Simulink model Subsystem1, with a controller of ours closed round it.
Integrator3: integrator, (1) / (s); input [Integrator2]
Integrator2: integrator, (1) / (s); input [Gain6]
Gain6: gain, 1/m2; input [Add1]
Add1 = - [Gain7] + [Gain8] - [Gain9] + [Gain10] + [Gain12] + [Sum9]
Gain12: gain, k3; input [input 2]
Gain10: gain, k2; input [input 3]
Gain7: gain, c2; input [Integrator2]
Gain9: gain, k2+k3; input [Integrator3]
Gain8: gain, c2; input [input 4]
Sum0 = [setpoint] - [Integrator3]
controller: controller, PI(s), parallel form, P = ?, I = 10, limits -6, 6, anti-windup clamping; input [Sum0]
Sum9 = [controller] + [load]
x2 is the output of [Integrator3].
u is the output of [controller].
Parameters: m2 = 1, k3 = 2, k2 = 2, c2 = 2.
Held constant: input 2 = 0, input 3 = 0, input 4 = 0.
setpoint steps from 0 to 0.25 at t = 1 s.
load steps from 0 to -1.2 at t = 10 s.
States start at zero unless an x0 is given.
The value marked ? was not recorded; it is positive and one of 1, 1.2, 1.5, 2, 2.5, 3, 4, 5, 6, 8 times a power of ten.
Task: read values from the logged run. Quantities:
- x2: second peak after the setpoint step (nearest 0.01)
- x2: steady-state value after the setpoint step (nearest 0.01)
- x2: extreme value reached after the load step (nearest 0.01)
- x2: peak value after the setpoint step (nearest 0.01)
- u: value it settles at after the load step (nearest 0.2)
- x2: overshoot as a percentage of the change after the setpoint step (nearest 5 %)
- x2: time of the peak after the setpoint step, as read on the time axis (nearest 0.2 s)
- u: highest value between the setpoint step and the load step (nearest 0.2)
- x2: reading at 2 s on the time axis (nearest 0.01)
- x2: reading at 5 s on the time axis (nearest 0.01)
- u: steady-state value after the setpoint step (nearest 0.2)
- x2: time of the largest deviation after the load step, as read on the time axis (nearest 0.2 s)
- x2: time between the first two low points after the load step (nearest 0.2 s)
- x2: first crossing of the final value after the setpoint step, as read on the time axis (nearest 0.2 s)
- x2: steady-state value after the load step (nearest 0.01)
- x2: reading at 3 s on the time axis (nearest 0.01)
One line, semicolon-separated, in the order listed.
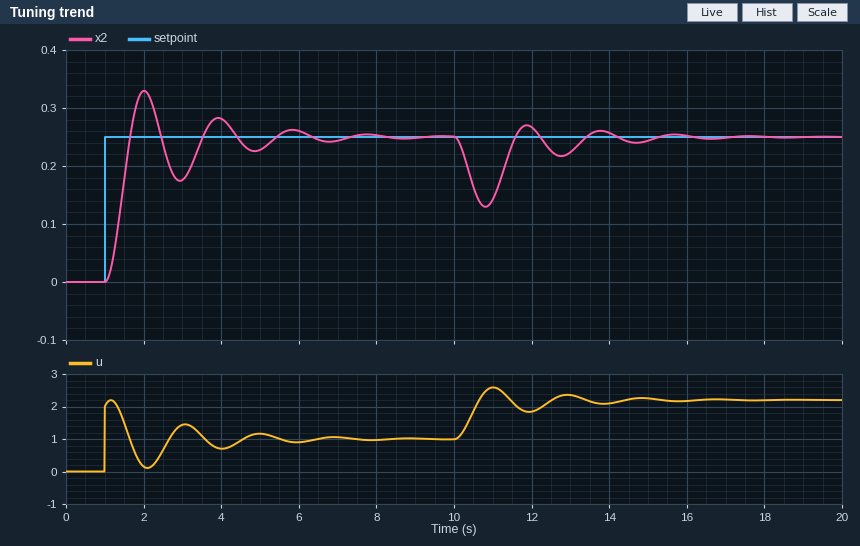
0.28; 0.25; 0.13; 0.33; 2.2; 30 %; 2.0 s; 2.2; 0.33; 0.23; 1.0; 10.8 s; 2.0 s; 1.6 s; 0.25; 0.18
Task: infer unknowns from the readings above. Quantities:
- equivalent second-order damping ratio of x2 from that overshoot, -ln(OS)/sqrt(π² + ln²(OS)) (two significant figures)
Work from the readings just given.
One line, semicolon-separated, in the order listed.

0.36
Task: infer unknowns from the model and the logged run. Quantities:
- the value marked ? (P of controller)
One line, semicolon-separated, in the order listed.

8
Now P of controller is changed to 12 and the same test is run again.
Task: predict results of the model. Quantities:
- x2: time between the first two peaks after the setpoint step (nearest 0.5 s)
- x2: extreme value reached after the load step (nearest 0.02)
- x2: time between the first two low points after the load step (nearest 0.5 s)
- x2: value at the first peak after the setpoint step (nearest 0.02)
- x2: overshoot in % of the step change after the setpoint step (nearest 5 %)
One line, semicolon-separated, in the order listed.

1.5 s; 0.16; 1.5 s; 0.34; 35 %
